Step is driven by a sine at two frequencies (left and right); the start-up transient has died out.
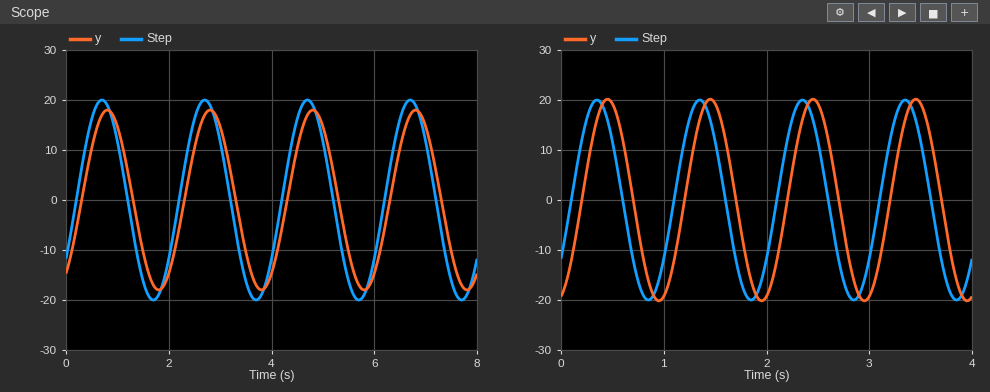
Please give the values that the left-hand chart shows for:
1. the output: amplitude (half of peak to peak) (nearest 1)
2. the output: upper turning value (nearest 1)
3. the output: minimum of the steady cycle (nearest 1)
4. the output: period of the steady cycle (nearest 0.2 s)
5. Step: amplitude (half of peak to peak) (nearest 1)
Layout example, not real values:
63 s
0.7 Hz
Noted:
18
18
-18
2.0 s
20
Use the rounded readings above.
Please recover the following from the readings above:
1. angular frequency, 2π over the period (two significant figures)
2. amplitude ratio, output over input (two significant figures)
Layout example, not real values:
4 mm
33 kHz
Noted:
3.1 rad/s
0.90
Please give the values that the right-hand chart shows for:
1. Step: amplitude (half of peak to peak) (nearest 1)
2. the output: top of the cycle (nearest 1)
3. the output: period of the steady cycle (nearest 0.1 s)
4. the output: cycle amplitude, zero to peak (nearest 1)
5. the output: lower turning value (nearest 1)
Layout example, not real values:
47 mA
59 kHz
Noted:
20
20
1.0 s
20
-20
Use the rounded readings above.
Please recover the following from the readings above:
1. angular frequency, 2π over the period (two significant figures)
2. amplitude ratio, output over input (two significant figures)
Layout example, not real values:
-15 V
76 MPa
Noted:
6.3 rad/s
1.0
